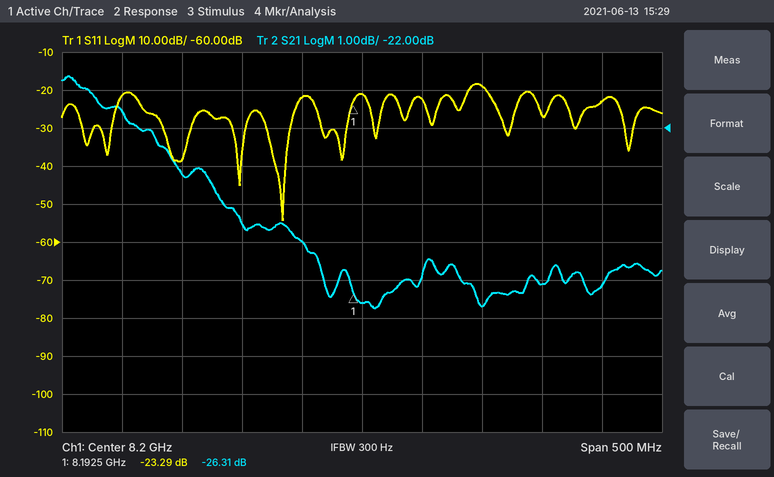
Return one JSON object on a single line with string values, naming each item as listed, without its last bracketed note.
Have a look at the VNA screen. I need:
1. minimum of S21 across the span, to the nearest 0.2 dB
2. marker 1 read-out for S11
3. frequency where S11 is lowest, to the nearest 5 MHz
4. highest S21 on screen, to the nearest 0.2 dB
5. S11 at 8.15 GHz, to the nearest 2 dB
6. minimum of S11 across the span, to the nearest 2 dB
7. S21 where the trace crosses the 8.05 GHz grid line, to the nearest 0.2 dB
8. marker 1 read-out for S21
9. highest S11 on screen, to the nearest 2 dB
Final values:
{"minimum of S21 across the span, to the nearest 0.2 dB": "-26.8 dB", "marker 1 read-out for S11": "-23.29 dB", "frequency where S11 is lowest, to the nearest 5 MHz": "8.135 GHz", "highest S21 on screen, to the nearest 0.2 dB": "-20.6 dB", "S11 at 8.15 GHz, to the nearest 2 dB": "-22 dB", "minimum of S11 across the span, to the nearest 2 dB": "-54 dB", "S21 where the trace crosses the 8.05 GHz grid line, to the nearest 0.2 dB": "-23.2 dB", "marker 1 read-out for S21": "-26.31 dB", "highest S11 on screen, to the nearest 2 dB": "-18 dB"}
